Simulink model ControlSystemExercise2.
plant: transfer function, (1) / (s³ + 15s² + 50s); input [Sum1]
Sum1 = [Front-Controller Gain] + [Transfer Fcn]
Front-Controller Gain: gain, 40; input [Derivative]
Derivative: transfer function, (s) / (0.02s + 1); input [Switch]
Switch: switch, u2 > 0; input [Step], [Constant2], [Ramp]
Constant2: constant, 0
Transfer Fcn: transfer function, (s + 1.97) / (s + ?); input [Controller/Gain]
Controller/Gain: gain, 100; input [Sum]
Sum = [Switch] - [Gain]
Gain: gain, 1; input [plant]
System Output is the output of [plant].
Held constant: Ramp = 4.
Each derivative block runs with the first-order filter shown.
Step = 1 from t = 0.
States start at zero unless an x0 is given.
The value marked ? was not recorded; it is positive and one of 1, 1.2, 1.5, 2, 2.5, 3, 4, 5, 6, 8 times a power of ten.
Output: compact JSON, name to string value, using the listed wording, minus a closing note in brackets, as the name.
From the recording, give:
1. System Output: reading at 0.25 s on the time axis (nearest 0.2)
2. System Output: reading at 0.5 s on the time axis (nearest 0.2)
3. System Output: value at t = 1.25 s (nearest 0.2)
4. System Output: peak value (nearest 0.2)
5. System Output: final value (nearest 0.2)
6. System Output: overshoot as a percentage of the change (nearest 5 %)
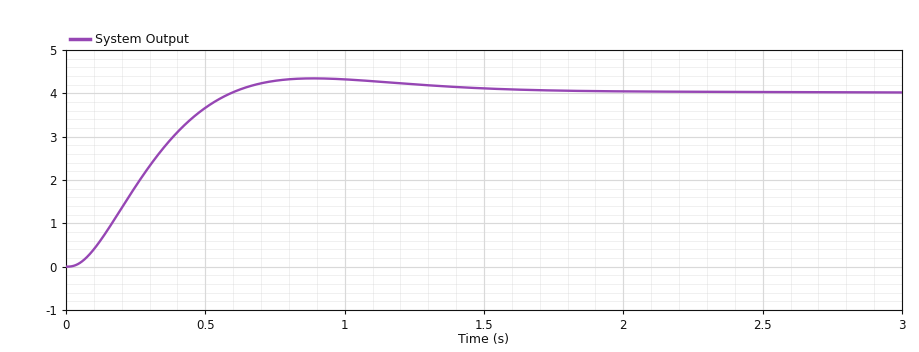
{"System Output: reading at 0.25 s on the time axis": "1.8", "System Output: reading at 0.5 s on the time axis": "3.6", "System Output: value at t = 1.25 s": "4.2", "System Output: peak value": "4.4", "System Output: final value": "4.0", "System Output: overshoot as a percentage of the change": "10 %"}
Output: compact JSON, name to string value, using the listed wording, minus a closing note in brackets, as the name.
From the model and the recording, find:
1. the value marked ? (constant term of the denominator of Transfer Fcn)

{"the value marked ?": "4"}
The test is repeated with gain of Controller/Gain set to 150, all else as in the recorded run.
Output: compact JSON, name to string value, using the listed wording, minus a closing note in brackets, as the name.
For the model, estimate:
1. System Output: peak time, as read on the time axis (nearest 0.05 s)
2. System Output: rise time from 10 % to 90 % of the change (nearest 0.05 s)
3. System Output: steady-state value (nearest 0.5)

{"System Output: peak time, as read on the time axis": "0.75 s", "System Output: rise time from 10 % to 90 % of the change": "0.30 s", "System Output: steady-state value": "4.0"}
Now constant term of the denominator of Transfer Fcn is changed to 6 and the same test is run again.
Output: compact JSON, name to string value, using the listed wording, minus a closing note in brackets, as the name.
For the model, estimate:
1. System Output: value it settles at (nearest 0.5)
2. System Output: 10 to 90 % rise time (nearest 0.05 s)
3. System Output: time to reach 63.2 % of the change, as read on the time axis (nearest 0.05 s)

{"System Output: value it settles at": "4.0", "System Output: 10 to 90 % rise time": "0.45 s", "System Output: time to reach 63.2 % of the change, as read on the time axis": "0.35 s"}
